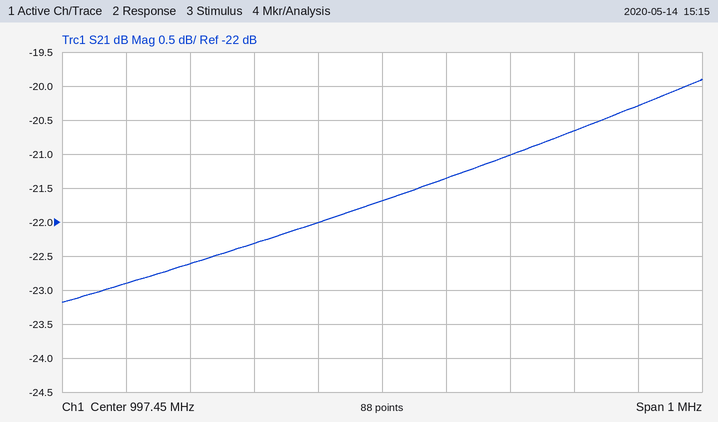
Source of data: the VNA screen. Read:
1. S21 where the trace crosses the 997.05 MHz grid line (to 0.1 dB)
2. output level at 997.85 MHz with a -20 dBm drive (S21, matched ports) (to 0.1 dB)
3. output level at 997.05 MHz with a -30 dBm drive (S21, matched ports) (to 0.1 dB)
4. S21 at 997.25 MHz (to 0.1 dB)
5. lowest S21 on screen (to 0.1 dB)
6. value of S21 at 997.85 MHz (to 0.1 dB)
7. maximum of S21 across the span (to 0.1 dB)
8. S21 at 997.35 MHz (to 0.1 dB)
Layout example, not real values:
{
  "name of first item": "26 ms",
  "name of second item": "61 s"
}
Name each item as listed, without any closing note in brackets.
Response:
{
  "S21 where the trace crosses the 997.05 MHz grid line": "-22.9 dB",
  "output level at 997.85 MHz with a -20 dBm drive (S21, matched ports)": "-40.3 dBm",
  "output level at 997.05 MHz with a -30 dBm drive (S21, matched ports)": "-52.9 dBm",
  "S21 at 997.25 MHz": "-22.3 dB",
  "lowest S21 on screen": "-23.2 dB",
  "value of S21 at 997.85 MHz": "-20.3 dB",
  "maximum of S21 across the span": "-19.9 dB",
  "S21 at 997.35 MHz": "-22.0 dB"
}
